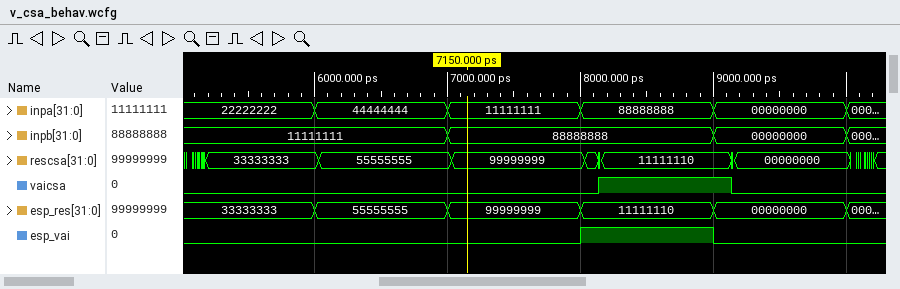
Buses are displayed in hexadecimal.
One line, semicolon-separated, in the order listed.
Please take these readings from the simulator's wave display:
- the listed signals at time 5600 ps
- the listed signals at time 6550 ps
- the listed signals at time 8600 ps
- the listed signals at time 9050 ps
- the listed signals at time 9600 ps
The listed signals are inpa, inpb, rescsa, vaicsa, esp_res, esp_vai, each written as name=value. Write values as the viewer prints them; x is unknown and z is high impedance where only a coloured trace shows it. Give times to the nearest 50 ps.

inpa=22222222, inpb=11111111, rescsa=33333333, vaicsa=0, esp_res=33333333, esp_vai=0; inpa=44444444, inpb=11111111, rescsa=55555555, vaicsa=0, esp_res=55555555, esp_vai=0; inpa=88888888, inpb=88888888, rescsa=11111110, vaicsa=1, esp_res=11111110, esp_vai=1; inpa=00000000, inpb=00000000, rescsa=11111110, vaicsa=1, esp_res=00000000, esp_vai=0; inpa=00000000, inpb=00000000, rescsa=00000000, vaicsa=0, esp_res=00000000, esp_vai=0
